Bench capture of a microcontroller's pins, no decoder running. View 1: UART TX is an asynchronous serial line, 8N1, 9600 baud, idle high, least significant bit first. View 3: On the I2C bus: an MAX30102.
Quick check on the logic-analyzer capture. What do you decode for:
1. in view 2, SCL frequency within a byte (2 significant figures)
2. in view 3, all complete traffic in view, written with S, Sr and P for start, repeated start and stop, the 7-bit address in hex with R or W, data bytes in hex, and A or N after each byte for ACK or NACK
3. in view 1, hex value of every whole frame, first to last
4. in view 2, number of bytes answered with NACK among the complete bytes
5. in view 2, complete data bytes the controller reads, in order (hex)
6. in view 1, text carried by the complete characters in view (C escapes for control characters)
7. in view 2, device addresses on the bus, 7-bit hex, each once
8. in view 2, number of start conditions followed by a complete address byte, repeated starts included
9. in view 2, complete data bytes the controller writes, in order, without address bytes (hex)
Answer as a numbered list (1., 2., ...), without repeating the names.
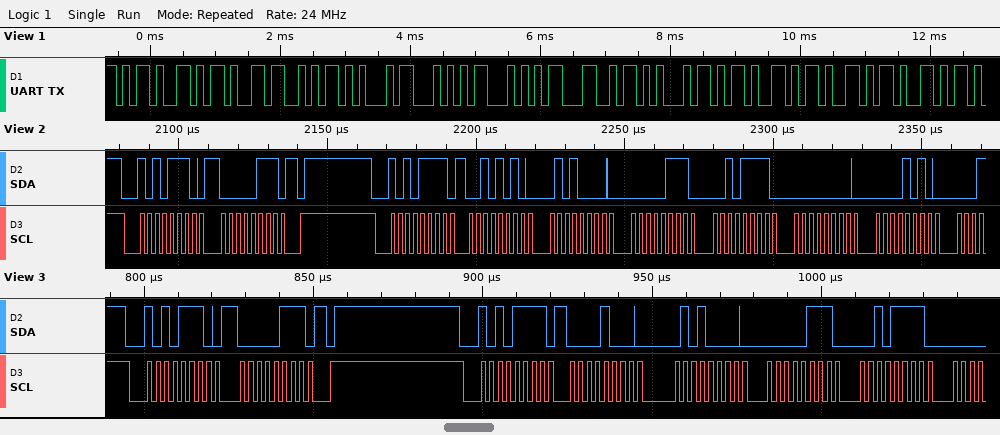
1. 400 kHz
2. S 57W A 07 A P S 57R A 08 A 50 A 07 A 2F A
3. 2D 2D 53 45 54 54 4C 45 2D 2D 2D
4. 0
5. 2A 50 07 2F 00 0A
6. "--SETTLE---"
7. 0x57
8. 2
9. 07
